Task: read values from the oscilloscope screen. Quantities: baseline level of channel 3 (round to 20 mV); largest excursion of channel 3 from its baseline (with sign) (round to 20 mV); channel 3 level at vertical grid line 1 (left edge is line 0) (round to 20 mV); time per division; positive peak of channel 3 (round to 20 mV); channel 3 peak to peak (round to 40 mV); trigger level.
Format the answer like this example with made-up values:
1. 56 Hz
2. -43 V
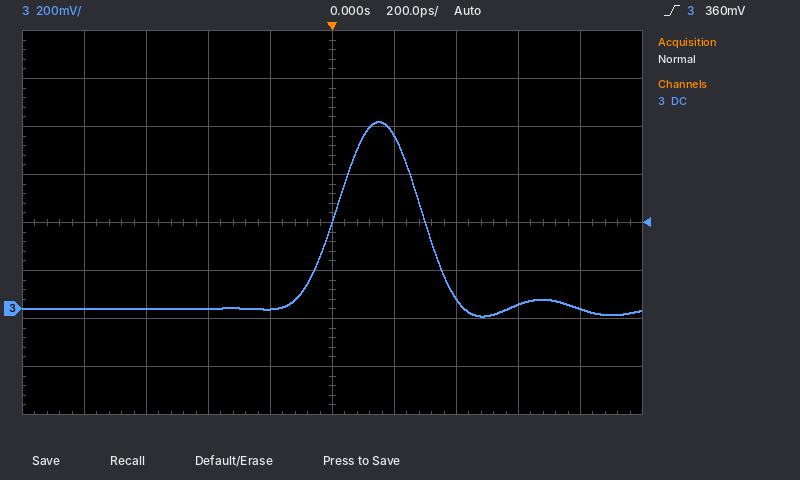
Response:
1. 0 mV
2. +780 mV
3. 0 mV
4. 200 ps
5. 780 mV
6. 800 mV
7. 360 mV
